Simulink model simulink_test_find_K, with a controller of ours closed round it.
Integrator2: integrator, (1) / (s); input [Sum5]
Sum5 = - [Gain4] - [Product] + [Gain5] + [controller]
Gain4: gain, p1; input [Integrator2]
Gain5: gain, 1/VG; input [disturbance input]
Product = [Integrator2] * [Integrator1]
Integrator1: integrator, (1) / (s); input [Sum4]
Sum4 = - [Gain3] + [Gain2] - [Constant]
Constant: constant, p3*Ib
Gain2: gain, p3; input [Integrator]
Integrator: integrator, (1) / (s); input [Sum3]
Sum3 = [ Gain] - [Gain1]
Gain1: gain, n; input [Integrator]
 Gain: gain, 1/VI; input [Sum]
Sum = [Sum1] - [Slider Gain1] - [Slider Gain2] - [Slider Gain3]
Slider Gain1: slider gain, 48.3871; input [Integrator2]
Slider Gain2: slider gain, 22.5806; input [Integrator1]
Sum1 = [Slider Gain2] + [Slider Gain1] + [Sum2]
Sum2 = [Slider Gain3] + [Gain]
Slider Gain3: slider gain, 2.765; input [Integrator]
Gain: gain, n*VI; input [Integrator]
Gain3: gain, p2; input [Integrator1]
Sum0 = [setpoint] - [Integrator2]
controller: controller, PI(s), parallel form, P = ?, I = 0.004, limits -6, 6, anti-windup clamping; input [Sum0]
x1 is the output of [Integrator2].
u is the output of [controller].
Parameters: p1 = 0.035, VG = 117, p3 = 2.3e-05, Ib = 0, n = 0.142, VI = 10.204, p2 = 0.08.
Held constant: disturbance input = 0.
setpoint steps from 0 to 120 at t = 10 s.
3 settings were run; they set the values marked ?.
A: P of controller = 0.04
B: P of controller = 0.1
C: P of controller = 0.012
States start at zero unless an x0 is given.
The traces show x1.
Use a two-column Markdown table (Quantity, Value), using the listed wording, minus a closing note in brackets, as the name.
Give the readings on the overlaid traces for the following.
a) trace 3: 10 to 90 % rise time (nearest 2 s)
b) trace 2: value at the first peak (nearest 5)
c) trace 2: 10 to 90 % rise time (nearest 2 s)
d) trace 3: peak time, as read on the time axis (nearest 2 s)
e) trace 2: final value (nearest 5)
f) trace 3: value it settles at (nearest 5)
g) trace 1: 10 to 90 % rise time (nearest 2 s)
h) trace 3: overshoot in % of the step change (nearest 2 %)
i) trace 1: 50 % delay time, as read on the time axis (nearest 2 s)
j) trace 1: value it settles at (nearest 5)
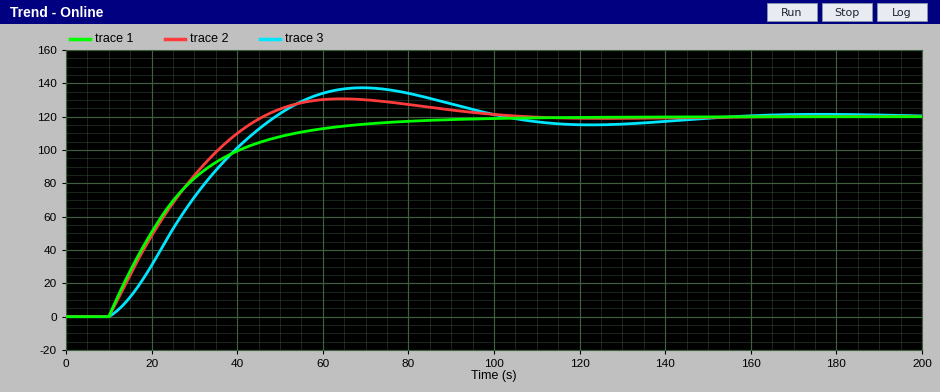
| Quantity | Value |
|---|---|
| trace 3: 10 to 90 % rise time | 28 s |
| trace 2: value at the first peak | 130 |
| trace 2: 10 to 90 % rise time | 26 s |
| trace 3: peak time, as read on the time axis | 70 s |
| trace 2: final value | 120 |
| trace 3: value it settles at | 120 |
| trace 1: 10 to 90 % rise time | 38 s |
| trace 3: overshoot in % of the step change | 14 % |
| trace 1: 50 % delay time, as read on the time axis | 22 s |
| trace 1: value it settles at | 120 |
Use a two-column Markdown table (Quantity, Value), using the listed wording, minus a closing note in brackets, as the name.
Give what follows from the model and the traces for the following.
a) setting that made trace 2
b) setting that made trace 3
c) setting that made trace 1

| Quantity | Value |
|---|---|
| setting that made trace 2 | A |
| setting that made trace 3 | C |
| setting that made trace 1 | B |
